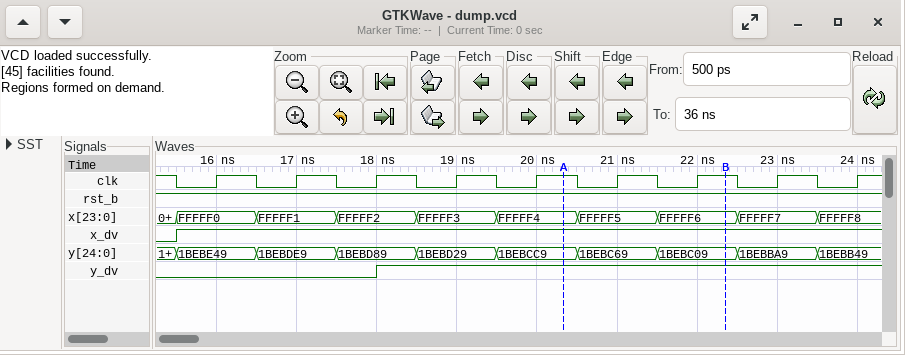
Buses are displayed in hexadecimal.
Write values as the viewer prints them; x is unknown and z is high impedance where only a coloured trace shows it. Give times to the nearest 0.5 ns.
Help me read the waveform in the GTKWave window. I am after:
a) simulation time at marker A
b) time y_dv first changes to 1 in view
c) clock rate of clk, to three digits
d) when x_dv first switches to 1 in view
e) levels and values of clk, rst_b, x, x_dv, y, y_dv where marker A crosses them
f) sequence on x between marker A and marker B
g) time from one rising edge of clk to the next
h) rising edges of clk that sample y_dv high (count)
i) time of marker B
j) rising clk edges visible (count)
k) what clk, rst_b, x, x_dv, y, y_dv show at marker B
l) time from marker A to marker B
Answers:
20.5 ns
18 ns
1.00 GHz
15.5 ns
clk=1, rst_b=1, x=FFFFF4, x_dv=1, y=1BEBCC9, y_dv=1
FFFFF4, FFFFF5, FFFFF6
1 ns
6
22.5 ns
9
clk=1, rst_b=1, x=FFFFF6, x_dv=1, y=1BEBC09, y_dv=1
2 ns
